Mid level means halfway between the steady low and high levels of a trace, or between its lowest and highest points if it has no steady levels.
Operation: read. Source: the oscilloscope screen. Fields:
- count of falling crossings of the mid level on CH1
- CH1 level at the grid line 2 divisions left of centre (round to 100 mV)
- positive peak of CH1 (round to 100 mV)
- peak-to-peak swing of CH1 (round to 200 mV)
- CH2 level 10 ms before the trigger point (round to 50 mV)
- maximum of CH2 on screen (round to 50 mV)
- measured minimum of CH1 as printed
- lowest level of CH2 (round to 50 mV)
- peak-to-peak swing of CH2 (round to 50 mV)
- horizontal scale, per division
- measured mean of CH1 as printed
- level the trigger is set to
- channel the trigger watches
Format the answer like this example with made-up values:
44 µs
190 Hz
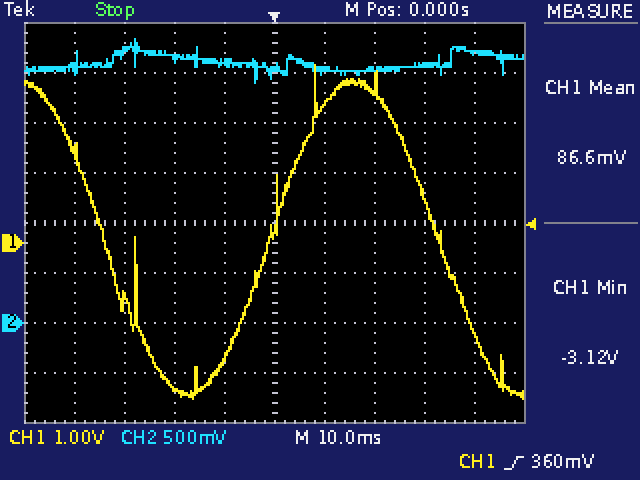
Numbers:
2
-2.9 V
3.6 V
6.6 V
2.60 V
2.85 V
-3.12 V
2.40 V
450 mV
10 ms
86.6 mV
360 mV
CH1
